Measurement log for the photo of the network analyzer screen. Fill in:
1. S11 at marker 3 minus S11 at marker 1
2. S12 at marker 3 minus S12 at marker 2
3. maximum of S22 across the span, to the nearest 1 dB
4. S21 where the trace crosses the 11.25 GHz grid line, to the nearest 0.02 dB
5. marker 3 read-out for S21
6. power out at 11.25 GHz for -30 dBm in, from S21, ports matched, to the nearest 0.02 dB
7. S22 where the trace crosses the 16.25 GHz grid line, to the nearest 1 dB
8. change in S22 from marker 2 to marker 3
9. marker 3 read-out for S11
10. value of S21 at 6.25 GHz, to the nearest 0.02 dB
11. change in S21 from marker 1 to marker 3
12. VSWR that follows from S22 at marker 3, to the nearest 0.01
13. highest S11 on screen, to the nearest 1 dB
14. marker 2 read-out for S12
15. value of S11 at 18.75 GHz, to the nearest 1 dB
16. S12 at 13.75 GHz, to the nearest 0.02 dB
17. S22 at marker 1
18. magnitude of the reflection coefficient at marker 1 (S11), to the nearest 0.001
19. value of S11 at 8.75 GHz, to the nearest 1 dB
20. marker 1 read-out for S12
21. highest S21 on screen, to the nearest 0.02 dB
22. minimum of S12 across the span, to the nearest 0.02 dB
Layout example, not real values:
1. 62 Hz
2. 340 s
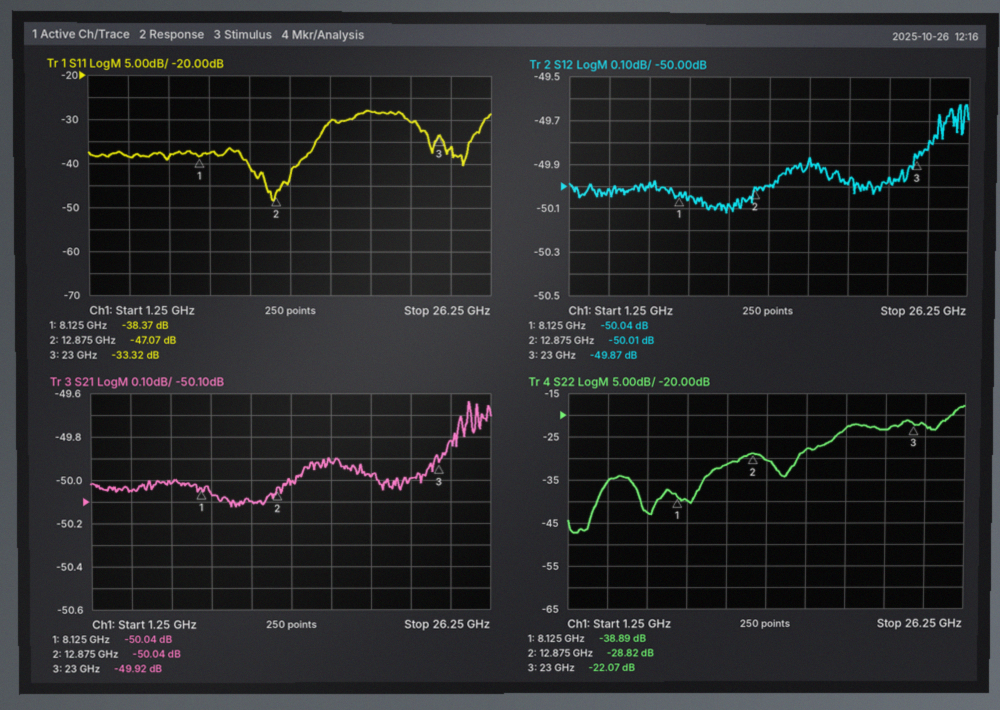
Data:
1. 5.05 dB
2. 0.14 dB
3. -18 dB
4. -50.10 dB
5. -49.92 dB
6. -80.10 dBm
7. -28 dB
8. 6.75 dB
9. -33.32 dB
10. -50.02 dB
11. 0.12 dB
12. 1.17
13. -28 dB
14. -50.01 dB
15. -28 dB
16. -50.00 dB
17. -38.89 dB
18. 0.012
19. -38 dB
20. -50.04 dB
21. -49.64 dB
22. -50.12 dB
